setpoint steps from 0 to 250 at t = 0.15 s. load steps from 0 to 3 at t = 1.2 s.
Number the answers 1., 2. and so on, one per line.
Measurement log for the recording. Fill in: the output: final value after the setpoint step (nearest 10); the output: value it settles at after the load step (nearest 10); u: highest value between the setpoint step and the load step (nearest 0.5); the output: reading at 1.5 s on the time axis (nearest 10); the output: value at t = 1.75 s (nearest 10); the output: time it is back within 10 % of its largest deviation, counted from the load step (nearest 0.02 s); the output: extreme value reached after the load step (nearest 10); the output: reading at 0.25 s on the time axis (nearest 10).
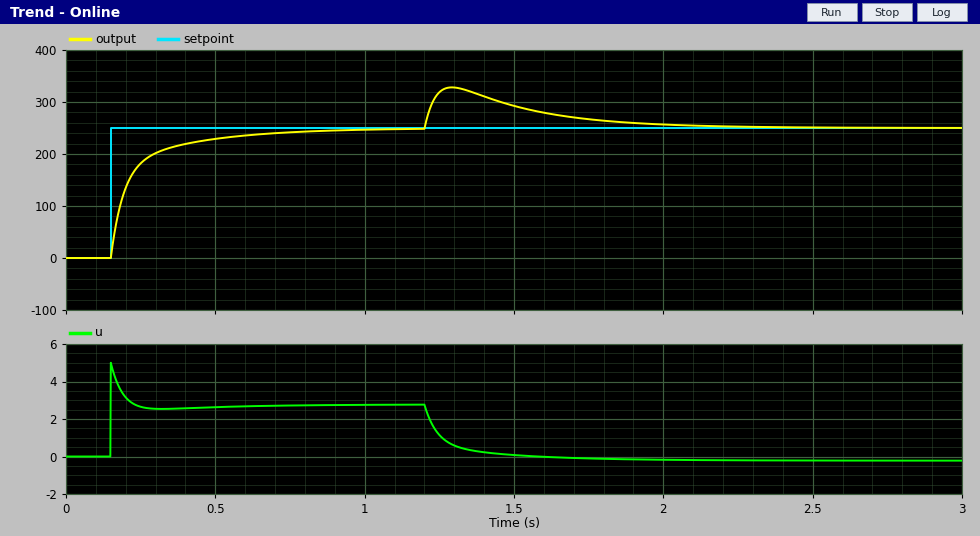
1. 250
2. 250
3. 5.0
4. 290
5. 270
6. 0.76 s
7. 330
8. 180
